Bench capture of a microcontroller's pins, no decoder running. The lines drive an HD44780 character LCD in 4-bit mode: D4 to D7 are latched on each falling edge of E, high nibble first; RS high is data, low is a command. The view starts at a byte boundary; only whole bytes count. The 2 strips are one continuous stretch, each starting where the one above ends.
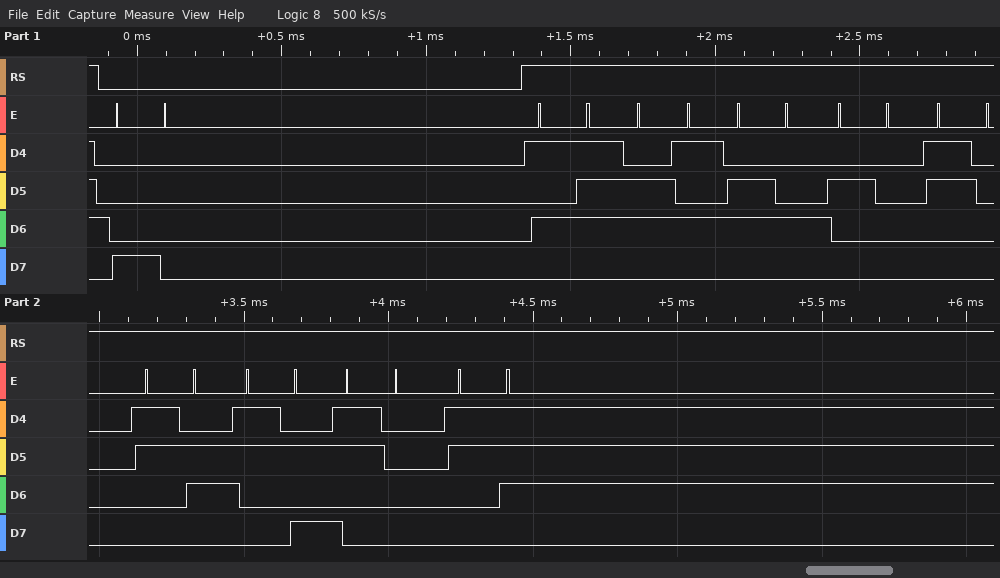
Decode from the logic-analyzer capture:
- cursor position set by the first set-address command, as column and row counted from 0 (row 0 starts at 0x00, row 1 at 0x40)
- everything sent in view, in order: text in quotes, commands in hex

column 0, row 0
0x80 "Wed 06:07"
